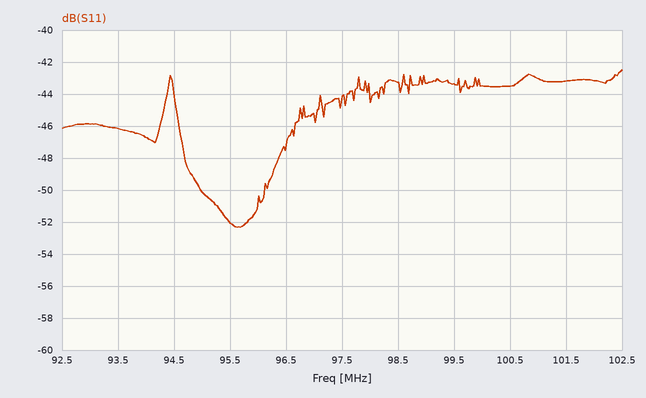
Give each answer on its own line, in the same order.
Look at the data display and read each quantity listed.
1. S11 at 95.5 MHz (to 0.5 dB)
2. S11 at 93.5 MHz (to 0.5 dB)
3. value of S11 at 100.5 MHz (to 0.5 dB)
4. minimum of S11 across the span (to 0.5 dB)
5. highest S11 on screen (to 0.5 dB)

-52.0 dB
-46.0 dB
-43.5 dB
-52.5 dB
-42.5 dB
